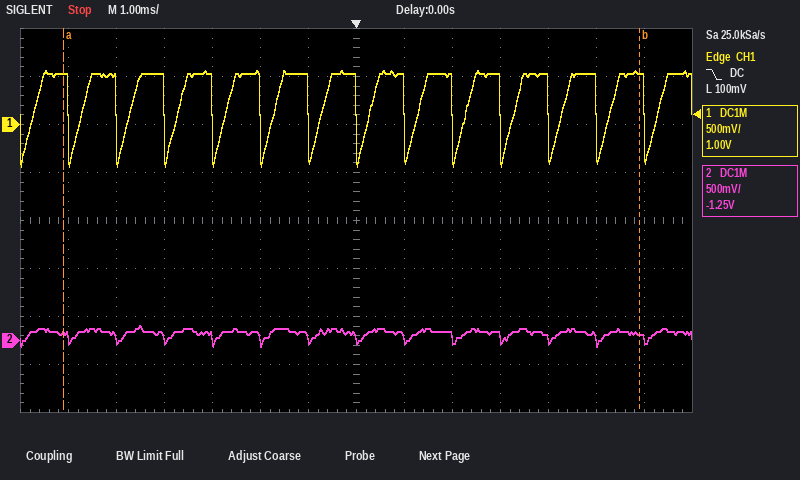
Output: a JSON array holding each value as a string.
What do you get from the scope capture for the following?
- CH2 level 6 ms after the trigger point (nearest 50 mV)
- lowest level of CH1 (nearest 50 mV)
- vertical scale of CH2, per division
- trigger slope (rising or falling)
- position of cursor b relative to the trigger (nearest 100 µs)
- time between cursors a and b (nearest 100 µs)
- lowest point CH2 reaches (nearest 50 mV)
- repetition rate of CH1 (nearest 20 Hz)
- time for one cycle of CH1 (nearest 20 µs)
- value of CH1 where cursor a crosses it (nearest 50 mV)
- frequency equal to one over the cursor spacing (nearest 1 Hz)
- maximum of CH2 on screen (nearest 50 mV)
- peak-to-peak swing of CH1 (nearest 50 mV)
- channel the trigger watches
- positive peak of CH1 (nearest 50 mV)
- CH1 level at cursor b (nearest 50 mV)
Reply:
["0 mV", "-450 mV", "500 mV", "falling", "+5.9 ms", "12.0 ms", "-50 mV", "1.00 kHz", "1.00 ms", "550 mV", "83 Hz", "150 mV", "1.00 V", "CH1", "550 mV", "550 mV"]
